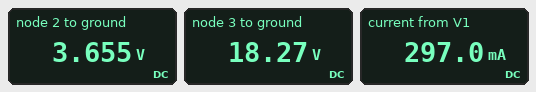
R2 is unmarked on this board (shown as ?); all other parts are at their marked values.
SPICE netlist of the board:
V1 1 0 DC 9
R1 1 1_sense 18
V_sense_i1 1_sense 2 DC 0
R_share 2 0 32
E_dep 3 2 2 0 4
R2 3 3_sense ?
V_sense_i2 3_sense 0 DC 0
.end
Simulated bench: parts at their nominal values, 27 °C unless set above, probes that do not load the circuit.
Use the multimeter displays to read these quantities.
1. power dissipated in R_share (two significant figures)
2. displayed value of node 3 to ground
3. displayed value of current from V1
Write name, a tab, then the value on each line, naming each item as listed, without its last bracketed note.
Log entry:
power dissipated in R_share	420 mW
displayed value of node 3 to ground	18.27 V
displayed value of current from V1	297.0 mA
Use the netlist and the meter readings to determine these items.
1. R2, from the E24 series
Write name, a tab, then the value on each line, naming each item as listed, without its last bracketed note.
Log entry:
R2, from the E24 series	100 Ω
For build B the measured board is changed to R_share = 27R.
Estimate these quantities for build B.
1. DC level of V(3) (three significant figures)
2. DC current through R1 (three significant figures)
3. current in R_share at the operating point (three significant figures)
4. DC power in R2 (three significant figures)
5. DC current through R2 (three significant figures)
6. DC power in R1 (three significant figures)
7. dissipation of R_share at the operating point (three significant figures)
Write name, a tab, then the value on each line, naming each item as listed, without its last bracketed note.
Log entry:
DC level of V(3)	17.5 V
DC current through R1	305 mA
current in R_share at the operating point	130 mA
DC power in R2	3.07 W
DC current through R2	175 mA
DC power in R1	1.68 W
dissipation of R_share at the operating point	455 mW
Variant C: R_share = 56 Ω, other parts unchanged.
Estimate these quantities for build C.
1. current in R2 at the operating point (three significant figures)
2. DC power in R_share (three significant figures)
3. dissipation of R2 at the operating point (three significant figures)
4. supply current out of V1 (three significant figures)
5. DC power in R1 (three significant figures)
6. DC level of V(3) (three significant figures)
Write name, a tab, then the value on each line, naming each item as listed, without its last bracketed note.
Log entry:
current in R2 at the operating point	203 mA
DC power in R_share	293 mW
dissipation of R2 at the operating point	4.10 W
supply current out of V1	275 mA
DC power in R1	1.36 W
DC level of V(3)	20.3 V
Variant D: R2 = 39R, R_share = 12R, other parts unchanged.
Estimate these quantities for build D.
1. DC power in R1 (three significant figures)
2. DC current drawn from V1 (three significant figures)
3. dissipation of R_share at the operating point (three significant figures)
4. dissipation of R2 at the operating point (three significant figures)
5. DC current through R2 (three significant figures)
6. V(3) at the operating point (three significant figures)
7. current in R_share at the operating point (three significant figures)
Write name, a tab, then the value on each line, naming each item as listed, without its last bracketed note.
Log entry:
DC power in R1	2.82 W
DC current drawn from V1	396 mA
dissipation of R_share at the operating point	292 mW
dissipation of R2 at the operating point	2.25 W
DC current through R2	240 mA
V(3) at the operating point	9.36 V
current in R_share at the operating point	156 mA
